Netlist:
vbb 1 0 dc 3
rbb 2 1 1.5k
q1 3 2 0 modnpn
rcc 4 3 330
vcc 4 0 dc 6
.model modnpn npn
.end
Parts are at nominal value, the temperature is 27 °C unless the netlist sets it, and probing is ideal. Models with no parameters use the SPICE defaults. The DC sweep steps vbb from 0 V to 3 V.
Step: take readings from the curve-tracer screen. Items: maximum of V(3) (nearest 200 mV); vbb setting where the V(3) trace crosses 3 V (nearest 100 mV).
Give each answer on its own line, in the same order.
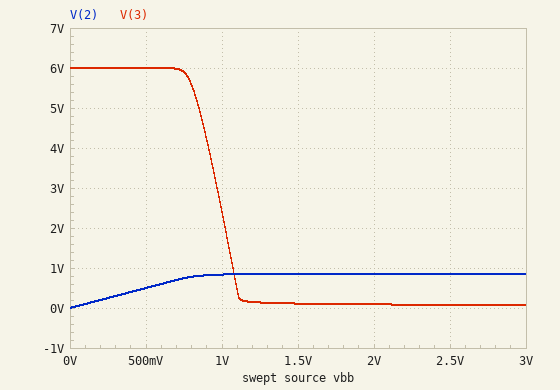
6.0 V
1.0 V
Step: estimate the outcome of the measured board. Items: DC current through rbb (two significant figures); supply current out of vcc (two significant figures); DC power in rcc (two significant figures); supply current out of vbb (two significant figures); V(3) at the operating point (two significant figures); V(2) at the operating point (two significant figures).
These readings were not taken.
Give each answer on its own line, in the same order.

1.4 mA
18 mA
110 mW
1.4 mA
73 mV
850 mV
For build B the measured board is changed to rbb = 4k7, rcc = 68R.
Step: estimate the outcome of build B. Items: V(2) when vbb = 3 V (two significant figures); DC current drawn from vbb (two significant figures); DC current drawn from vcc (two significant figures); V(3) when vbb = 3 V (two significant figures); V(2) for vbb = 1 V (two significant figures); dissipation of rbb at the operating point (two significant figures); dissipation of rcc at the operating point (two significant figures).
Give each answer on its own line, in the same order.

870 mV
450 µA
45 mA
2.9 V
810 mV
960 µW
140 mW
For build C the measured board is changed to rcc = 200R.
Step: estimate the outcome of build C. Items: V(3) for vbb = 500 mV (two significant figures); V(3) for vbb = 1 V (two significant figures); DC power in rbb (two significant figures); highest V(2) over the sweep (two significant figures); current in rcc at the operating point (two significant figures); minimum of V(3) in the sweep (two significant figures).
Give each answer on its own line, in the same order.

6.0 V
3.8 V
3.0 mW
860 mV
30 mA
87 mV
